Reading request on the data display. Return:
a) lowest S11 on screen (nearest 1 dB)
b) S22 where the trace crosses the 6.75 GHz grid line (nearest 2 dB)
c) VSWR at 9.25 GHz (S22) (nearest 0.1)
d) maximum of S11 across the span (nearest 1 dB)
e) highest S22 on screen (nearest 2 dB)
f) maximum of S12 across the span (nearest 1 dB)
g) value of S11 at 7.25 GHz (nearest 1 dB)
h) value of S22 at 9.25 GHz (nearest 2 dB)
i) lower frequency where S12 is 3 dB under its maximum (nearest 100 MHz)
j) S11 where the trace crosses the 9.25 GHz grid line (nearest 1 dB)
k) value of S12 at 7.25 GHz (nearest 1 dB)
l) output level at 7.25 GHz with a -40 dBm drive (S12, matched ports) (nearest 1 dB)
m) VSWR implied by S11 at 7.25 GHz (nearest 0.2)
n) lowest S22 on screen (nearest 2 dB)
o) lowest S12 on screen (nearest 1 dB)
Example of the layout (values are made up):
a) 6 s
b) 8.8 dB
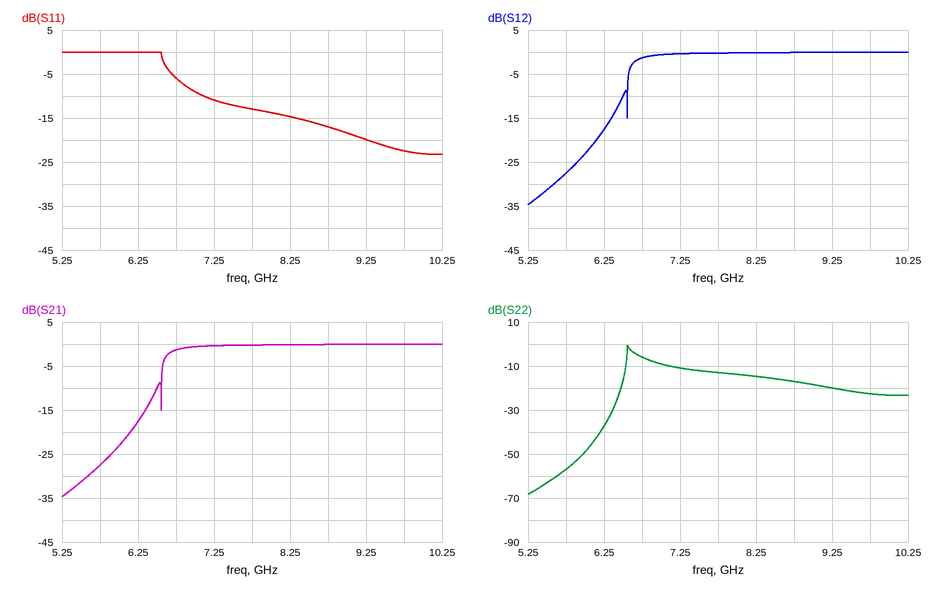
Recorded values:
a) -23 dB
b) -6 dB
c) 1.2
d) 0 dB
e) 0 dB
f) 0 dB
g) -11 dB
h) -20 dB
i) 6.6 GHz
j) -20 dB
k) 0 dB
l) -40 dBm
m) 1.8
n) -68 dB
o) -35 dB
